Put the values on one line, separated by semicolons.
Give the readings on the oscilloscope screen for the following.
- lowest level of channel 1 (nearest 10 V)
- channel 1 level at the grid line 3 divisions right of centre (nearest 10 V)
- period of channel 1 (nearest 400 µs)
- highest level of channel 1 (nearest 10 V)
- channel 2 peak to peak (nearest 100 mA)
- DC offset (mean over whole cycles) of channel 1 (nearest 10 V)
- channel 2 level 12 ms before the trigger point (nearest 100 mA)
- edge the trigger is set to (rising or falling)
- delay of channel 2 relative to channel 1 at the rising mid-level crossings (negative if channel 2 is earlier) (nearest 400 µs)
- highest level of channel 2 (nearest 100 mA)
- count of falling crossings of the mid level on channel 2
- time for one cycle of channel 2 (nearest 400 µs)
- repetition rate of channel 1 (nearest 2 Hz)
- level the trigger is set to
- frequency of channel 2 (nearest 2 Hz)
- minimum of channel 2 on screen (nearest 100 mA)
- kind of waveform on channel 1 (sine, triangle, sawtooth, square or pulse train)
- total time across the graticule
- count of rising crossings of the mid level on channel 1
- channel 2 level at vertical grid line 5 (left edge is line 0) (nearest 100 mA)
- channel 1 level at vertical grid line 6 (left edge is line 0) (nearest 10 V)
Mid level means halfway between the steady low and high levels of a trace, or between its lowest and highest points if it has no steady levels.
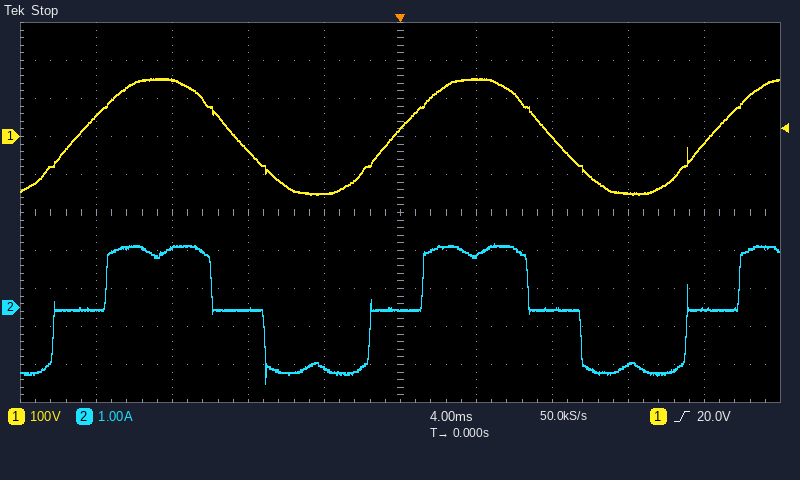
-150 V; -150 V; 16.8 ms; 150 V; 3.7 A; 0 V; 1.6 A; rising; -1.2 ms; 1.7 A; 2; 16.8 ms; 60 Hz; 20.0 V; 60 Hz; -2.0 A; sine; 40 ms; 3; -100 mA; 150 V
